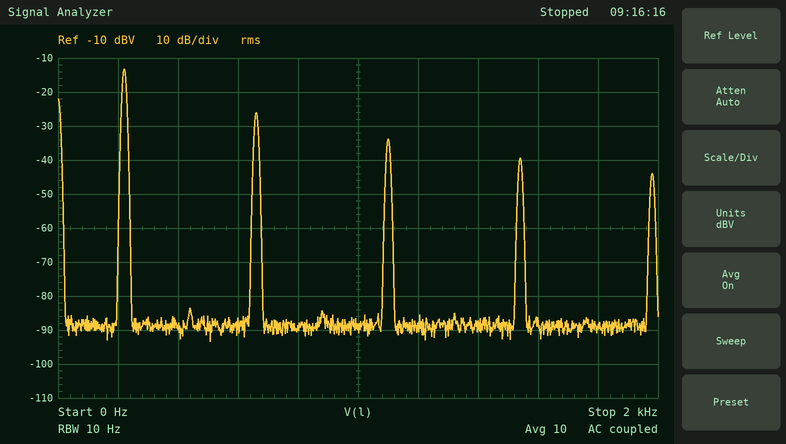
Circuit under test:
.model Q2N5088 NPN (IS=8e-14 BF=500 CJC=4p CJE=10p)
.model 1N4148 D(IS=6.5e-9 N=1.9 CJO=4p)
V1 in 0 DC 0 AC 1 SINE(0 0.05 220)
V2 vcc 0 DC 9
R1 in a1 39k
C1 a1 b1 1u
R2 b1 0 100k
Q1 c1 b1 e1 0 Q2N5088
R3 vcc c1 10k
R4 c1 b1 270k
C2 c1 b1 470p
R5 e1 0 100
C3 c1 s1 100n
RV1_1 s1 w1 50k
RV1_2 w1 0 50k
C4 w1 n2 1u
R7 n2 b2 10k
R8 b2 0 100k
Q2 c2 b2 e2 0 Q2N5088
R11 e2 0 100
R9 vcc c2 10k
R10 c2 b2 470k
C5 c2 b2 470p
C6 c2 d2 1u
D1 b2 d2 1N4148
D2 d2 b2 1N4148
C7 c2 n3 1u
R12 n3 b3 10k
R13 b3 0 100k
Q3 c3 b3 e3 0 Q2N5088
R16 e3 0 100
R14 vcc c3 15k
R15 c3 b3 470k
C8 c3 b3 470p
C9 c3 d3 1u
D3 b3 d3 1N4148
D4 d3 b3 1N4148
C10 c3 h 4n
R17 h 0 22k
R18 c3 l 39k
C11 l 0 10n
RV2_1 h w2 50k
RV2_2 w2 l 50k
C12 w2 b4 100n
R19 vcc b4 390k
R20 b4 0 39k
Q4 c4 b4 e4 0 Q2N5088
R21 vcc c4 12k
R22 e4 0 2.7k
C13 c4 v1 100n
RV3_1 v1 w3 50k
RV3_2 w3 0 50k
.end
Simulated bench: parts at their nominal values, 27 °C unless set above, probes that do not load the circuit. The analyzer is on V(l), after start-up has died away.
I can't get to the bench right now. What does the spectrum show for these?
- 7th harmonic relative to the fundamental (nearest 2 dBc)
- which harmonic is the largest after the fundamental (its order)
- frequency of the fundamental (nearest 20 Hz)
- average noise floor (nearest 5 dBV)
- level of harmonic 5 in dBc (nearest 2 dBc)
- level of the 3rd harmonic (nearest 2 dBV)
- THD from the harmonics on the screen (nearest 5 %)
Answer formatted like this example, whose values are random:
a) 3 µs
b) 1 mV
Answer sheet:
a) -26 dBc
b) 3
c) 220 Hz
d) -90 dBV
e) -20 dBc
f) -26 dBV
g) 25 %
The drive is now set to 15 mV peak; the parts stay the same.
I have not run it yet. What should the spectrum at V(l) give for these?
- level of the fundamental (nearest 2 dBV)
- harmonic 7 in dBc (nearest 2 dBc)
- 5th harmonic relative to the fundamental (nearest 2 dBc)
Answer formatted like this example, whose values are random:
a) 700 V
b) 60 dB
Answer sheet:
a) -14 dBV
b) -28 dBc
c) -22 dBc
